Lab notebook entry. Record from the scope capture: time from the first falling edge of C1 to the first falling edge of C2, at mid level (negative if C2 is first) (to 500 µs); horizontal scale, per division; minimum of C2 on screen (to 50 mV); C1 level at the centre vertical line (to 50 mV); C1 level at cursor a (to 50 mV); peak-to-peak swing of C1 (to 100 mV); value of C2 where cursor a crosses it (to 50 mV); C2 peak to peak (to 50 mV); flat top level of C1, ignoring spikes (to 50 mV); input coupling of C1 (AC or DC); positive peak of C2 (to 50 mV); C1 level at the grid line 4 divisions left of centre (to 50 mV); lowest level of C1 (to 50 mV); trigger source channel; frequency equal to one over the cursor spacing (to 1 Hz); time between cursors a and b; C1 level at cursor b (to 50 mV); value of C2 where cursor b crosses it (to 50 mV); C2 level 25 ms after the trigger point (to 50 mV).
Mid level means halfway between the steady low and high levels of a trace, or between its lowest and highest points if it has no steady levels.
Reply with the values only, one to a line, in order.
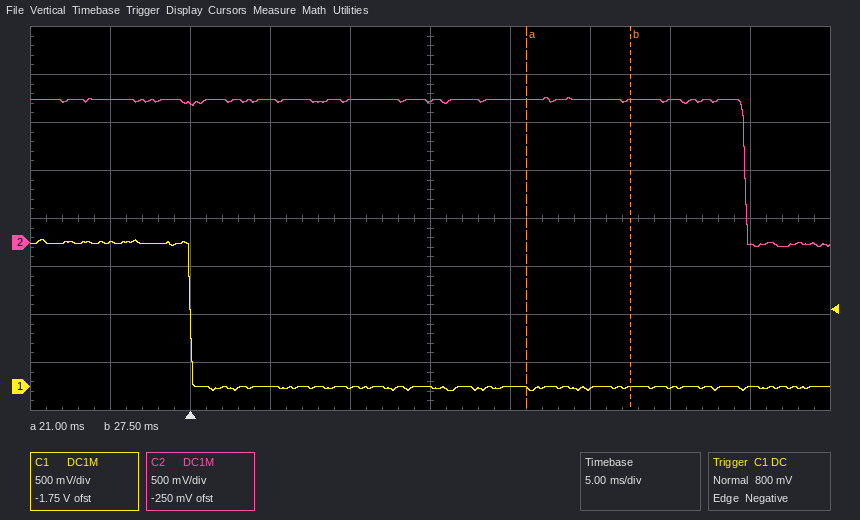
+34.5 ms
5 ms
-50 mV
0 mV
0 mV
1.60 V
1.50 V
1.55 V
1.50 V
DC
1.50 V
1.50 V
-50 mV
C1
154 Hz
6.5 ms
0 mV
1.50 V
1.50 V
